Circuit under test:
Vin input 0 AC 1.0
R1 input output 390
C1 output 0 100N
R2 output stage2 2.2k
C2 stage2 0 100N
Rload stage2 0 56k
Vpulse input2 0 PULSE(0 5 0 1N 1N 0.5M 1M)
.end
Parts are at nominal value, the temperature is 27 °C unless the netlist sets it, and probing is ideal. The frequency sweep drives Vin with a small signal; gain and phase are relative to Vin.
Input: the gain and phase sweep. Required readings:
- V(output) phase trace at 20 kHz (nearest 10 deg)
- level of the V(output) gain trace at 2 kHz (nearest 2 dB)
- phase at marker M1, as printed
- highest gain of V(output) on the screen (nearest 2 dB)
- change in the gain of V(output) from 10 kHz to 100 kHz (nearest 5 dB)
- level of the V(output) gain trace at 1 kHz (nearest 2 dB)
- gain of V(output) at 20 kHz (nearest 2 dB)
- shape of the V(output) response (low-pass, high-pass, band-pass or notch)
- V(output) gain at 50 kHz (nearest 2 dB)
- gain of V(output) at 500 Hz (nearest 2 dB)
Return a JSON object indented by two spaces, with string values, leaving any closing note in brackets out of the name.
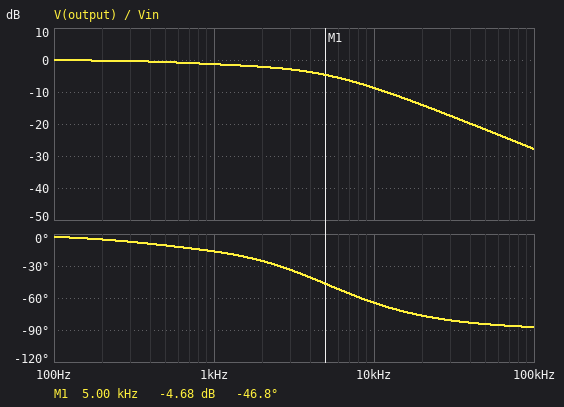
{
  "V(output) phase trace at 20 kHz": "-80 deg",
  "level of the V(output) gain trace at 2 kHz": "-2 dB",
  "phase at marker M1, as printed": "-46.8 deg",
  "highest gain of V(output) on the screen": "0 dB",
  "change in the gain of V(output) from 10 kHz to 100 kHz": "-20 dB",
  "level of the V(output) gain trace at 1 kHz": "-2 dB",
  "gain of V(output) at 20 kHz": "-14 dB",
  "shape of the V(output) response": "low-pass",
  "V(output) gain at 50 kHz": "-22 dB",
  "gain of V(output) at 500 Hz": "0 dB"
}
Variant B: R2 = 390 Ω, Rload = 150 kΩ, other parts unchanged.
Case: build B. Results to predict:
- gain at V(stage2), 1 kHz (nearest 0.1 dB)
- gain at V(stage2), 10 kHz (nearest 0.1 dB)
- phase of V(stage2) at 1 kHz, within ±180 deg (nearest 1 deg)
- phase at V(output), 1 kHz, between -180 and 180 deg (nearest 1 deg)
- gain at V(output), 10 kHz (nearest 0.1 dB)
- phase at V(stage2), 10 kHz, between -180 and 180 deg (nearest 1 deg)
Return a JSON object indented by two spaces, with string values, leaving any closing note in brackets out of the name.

{
  "gain at V(stage2), 1 kHz": "-1.6 dB",
  "gain at V(stage2), 10 kHz": "-19.0 dB",
  "phase of V(stage2) at 1 kHz, within ±180 deg": "-38 deg",
  "phase at V(output), 1 kHz, between -180 and 180 deg": "-24 deg",
  "gain at V(output), 10 kHz": "-10.5 dB",
  "phase at V(stage2), 10 kHz, between -180 and 180 deg": "-124 deg"
}
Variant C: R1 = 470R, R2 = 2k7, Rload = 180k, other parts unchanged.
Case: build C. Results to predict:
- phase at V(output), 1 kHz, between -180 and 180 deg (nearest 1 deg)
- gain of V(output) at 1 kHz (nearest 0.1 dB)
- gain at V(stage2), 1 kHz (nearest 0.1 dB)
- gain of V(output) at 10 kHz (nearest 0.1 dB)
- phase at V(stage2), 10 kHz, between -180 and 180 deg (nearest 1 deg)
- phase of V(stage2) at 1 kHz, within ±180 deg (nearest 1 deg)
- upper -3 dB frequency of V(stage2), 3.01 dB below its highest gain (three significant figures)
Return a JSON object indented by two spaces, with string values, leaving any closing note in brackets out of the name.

{
  "phase at V(output), 1 kHz, between -180 and 180 deg": "-18 deg",
  "gain of V(output) at 1 kHz": "-1.5 dB",
  "gain at V(stage2), 1 kHz": "-7.4 dB",
  "gain of V(output) at 10 kHz": "-10.1 dB",
  "phase at V(stage2), 10 kHz, between -180 and 180 deg": "-155 deg",
  "phase of V(stage2) at 1 kHz, within ±180 deg": "-77 deg",
  "upper -3 dB frequency of V(stage2), 3.01 dB below its highest gain": "491 Hz"
}
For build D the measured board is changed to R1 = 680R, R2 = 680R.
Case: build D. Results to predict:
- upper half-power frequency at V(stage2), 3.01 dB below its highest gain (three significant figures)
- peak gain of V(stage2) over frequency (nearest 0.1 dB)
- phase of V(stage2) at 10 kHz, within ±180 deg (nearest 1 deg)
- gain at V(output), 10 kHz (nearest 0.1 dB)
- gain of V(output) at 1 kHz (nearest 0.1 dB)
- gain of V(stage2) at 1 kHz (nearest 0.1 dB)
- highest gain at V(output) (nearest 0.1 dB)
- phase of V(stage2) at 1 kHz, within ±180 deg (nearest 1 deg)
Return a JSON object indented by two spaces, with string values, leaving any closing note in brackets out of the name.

{
  "upper half-power frequency at V(stage2), 3.01 dB below its highest gain": "895 Hz",
  "peak gain of V(stage2) over frequency": "-0.2 dB",
  "phase of V(stage2) at 10 kHz, within ±180 deg": "-143 deg",
  "gain at V(output), 10 kHz": "-13.8 dB",
  "gain of V(output) at 1 kHz": "-2.9 dB",
  "gain of V(stage2) at 1 kHz": "-3.7 dB",
  "highest gain at V(output)": "-0.1 dB",
  "phase of V(stage2) at 1 kHz, within ±180 deg": "-57 deg"
}
